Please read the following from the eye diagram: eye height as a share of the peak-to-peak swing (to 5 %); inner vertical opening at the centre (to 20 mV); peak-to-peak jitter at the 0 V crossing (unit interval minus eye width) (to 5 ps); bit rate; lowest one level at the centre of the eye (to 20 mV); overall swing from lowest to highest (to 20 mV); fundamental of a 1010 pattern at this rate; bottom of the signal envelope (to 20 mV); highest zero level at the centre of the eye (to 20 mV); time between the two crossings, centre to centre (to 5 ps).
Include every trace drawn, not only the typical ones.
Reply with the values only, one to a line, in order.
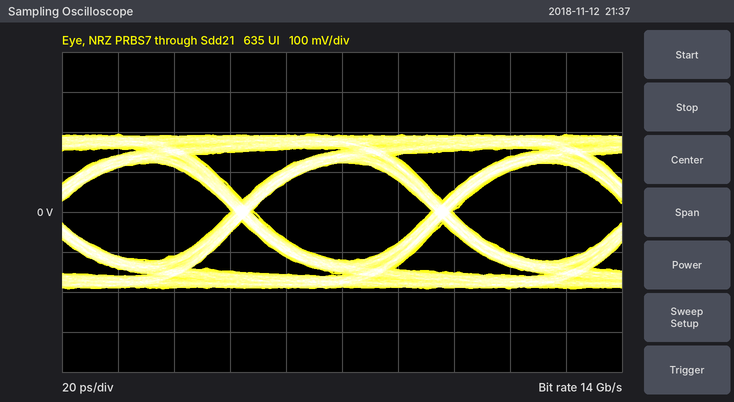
65 %
240 mV
10 ps
14 Gb/s
120 mV
380 mV
7 GHz
-200 mV
-120 mV
70 ps
